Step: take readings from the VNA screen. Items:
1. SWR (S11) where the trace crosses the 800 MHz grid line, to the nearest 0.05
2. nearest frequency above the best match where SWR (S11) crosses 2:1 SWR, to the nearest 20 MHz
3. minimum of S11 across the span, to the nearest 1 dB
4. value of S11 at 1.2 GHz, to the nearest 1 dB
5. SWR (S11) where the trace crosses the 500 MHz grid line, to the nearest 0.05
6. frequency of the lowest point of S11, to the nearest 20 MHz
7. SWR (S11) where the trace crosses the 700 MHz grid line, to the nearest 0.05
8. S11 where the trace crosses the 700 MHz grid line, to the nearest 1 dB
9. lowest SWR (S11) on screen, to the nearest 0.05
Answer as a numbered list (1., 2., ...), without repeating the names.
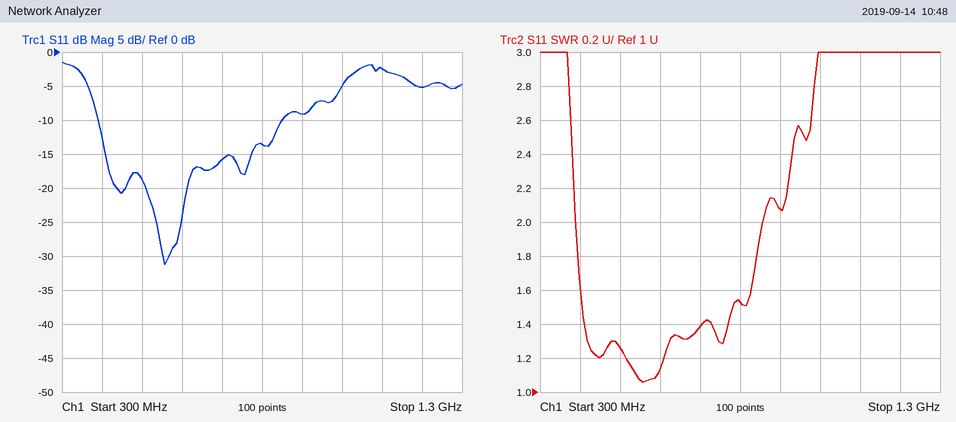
1. 1.55
2. 860 MHz
3. -31 dB
4. -5 dB
5. 1.25
6. 560 MHz
7. 1.40
8. -16 dB
9. 1.05
